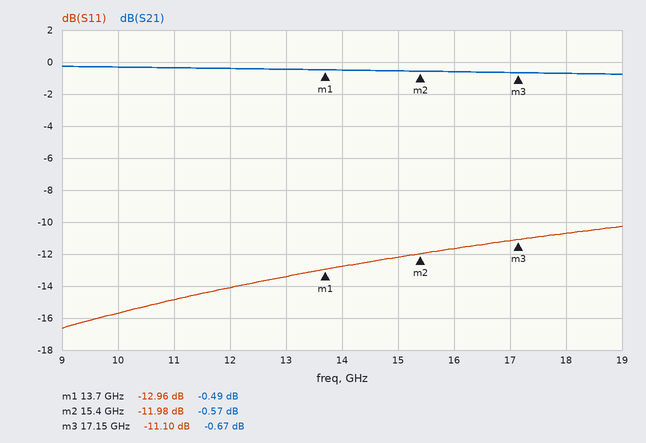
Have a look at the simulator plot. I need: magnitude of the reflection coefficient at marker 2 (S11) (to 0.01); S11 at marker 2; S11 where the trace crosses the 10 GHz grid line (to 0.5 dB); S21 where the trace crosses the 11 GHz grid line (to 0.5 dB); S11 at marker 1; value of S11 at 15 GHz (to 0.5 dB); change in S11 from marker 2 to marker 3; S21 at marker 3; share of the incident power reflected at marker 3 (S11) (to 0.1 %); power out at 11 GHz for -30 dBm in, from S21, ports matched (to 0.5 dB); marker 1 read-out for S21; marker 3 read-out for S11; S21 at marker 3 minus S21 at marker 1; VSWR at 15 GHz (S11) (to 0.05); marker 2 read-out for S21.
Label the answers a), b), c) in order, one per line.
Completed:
a) 0.25
b) -11.98 dB
c) -15.5 dB
d) -0.5 dB
e) -12.96 dB
f) -12.0 dB
g) 0.88 dB
h) -0.67 dB
i) 7.8 %
j) -30.5 dBm
k) -0.49 dB
l) -11.10 dB
m) -0.18 dB
n) 1.65
o) -0.57 dB
